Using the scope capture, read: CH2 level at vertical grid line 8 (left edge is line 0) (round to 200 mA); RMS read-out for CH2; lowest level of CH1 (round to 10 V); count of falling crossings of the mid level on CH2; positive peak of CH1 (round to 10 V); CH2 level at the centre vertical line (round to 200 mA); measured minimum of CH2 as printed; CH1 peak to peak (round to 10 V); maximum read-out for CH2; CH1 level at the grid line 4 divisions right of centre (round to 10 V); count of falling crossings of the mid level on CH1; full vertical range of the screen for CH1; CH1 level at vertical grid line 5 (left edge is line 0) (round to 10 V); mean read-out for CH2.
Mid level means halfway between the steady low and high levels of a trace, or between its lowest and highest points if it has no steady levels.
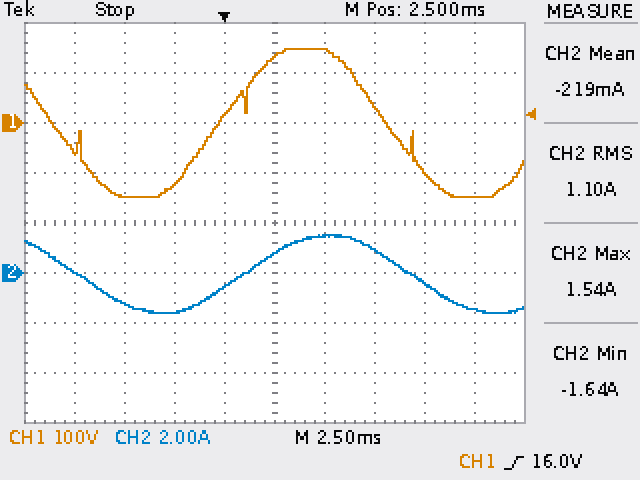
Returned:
-400 mA
1.10 A
-150 V
2
150 V
800 mA
-1.64 A
300 V
1.54 A
-150 V
2
800 V
130 V
-219 mA
